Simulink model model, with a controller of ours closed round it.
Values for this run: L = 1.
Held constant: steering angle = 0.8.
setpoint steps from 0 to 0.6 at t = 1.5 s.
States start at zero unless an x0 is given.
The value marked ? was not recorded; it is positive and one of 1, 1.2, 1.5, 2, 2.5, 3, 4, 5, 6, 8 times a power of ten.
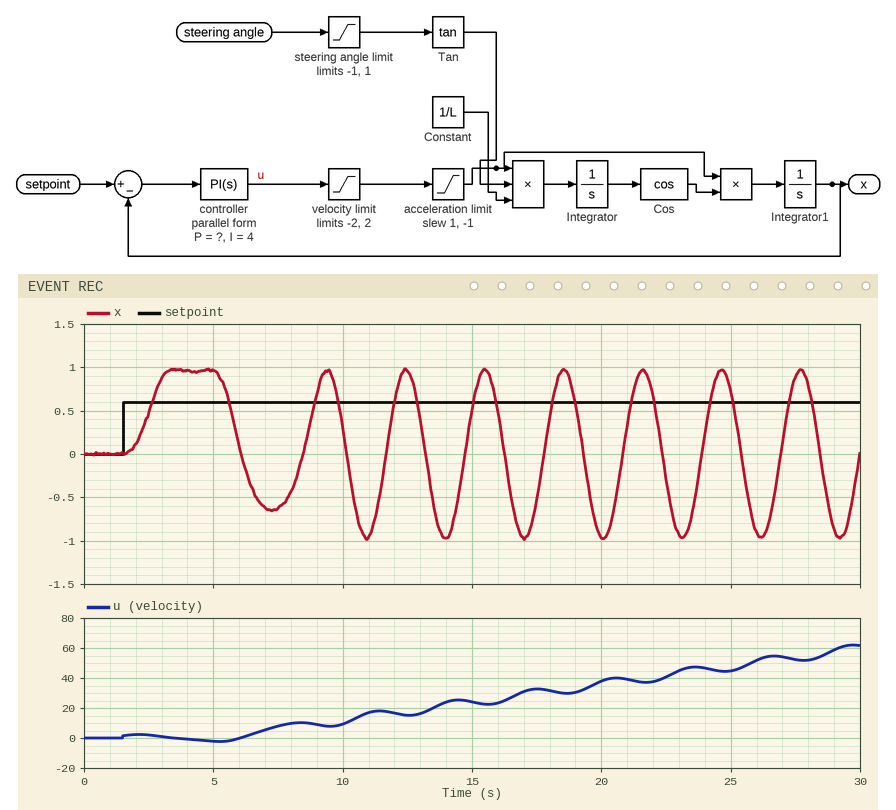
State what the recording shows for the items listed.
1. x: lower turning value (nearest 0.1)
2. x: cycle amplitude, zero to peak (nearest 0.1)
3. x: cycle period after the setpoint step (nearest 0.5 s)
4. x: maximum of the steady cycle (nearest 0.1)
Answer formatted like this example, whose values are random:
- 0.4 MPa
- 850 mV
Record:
- -1.0
- 1.0
- 3.0 s
- 1.0
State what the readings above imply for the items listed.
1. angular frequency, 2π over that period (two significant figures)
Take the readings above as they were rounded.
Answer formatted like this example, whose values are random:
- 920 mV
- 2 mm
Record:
- 2.1 rad/s
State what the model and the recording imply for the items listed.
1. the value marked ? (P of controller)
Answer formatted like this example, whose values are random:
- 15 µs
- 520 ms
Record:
- 2.5
